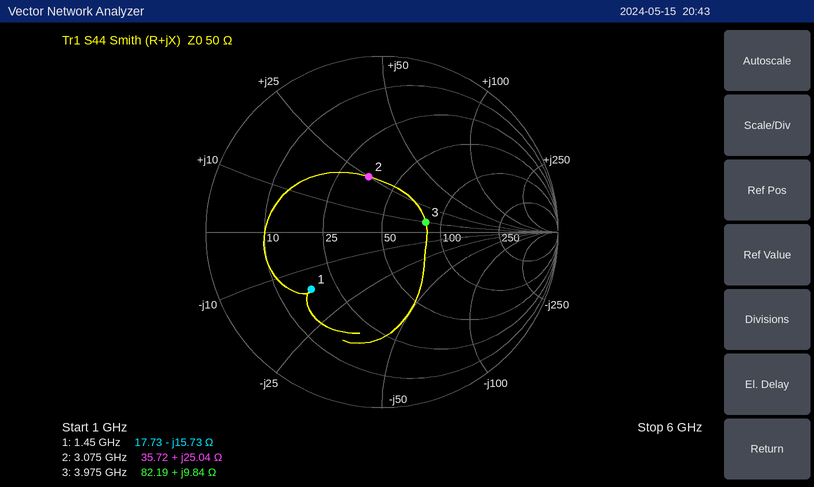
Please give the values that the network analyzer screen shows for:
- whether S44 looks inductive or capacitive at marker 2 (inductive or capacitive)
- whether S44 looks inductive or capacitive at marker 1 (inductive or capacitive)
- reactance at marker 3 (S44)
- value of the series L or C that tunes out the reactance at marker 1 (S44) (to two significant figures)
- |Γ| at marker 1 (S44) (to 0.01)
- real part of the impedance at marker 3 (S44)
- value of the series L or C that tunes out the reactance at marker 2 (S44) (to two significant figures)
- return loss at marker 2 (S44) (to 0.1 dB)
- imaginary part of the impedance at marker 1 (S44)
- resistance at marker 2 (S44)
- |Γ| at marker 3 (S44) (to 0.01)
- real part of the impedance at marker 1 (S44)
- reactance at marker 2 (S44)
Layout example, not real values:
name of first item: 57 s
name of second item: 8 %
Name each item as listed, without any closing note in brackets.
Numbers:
whether S44 looks inductive or capacitive at marker 2: inductive
whether S44 looks inductive or capacitive at marker 1: capacitive
reactance at marker 3: +9.84 Ω
value of the series L or C that tunes out the reactance at marker 1 (S44): 1.7 nH
|Γ| at marker 1 (S44): 0.52
real part of the impedance at marker 3: 82.19 Ω
value of the series L or C that tunes out the reactance at marker 2 (S44): 2.1 pF
return loss at marker 2 (S44): 9.8 dB
imaginary part of the impedance at marker 1: -15.73 Ω
resistance at marker 2: 35.72 Ω
|Γ| at marker 3 (S44): 0.25
real part of the impedance at marker 1: 17.73 Ω
reactance at marker 2: +25.04 Ω
